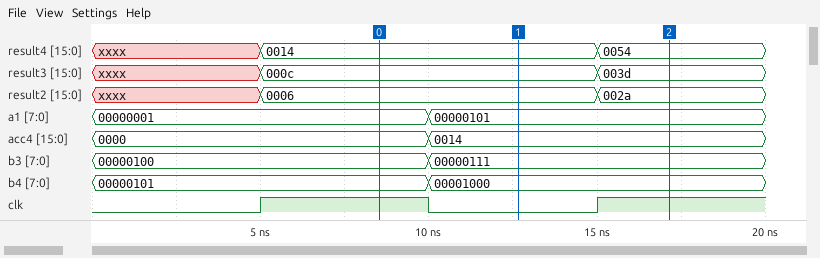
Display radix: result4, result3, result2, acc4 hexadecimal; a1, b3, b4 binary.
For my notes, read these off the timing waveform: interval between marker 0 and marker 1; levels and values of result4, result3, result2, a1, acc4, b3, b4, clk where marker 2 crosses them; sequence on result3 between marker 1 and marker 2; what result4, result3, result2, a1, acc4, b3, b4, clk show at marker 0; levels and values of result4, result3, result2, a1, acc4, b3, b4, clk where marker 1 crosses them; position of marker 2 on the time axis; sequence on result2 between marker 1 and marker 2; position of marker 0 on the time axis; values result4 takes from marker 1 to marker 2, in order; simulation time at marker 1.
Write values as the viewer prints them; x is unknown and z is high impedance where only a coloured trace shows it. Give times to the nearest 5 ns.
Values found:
5 ns
result4=0054, result3=003d, result2=002a, a1=00000101, acc4=0014, b3=00000111, b4=00001000, clk=1
000c, 003d
result4=0014, result3=000c, result2=0006, a1=00000001, acc4=0000, b3=00000100, b4=00000101, clk=1
result4=0014, result3=000c, result2=0006, a1=00000101, acc4=0014, b3=00000111, b4=00001000, clk=0
15 ns
0006, 002a
10 ns
0014, 0054
15 ns
